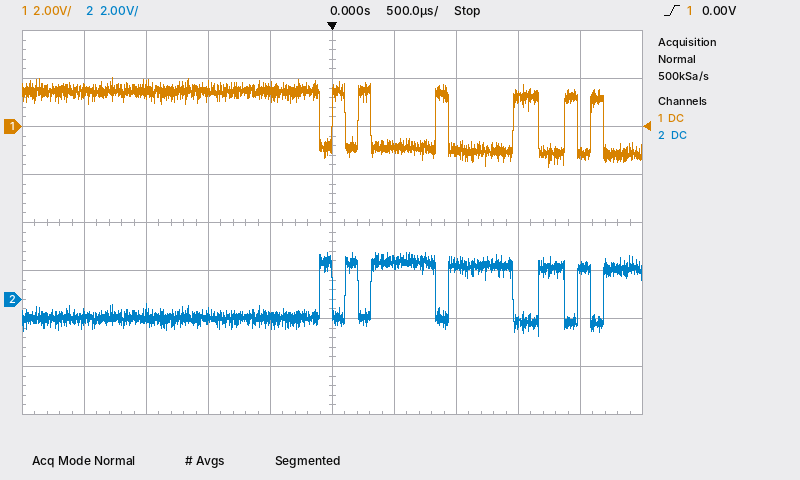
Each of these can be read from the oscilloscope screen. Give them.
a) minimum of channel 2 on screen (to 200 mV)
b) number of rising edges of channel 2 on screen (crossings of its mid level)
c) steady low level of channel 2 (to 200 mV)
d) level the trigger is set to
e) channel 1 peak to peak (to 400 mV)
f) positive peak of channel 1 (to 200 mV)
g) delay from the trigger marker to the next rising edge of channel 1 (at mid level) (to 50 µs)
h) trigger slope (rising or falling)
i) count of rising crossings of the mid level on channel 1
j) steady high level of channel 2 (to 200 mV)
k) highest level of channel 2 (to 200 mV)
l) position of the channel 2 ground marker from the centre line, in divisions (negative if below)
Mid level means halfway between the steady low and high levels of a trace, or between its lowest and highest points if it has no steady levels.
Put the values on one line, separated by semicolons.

-1.6 V; 7; -800 mV; 0.00 V; 3.6 V; 2.0 V; 200 µs; rising; 6; 1.4 V; 2.0 V; -1.6 div
